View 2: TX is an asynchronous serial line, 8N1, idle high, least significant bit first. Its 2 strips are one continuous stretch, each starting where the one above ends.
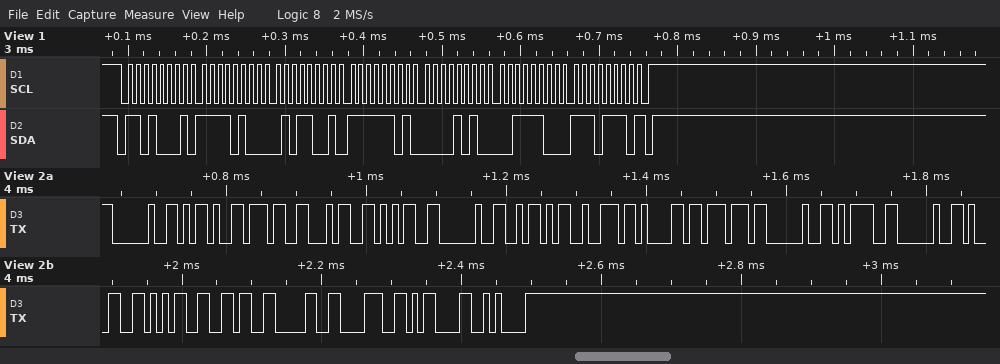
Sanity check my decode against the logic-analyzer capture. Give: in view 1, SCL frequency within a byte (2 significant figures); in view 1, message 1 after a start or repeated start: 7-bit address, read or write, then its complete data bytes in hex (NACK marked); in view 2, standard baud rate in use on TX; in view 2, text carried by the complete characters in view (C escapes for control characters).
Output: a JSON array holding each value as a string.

["100 kHz", "0x68 read: F4 59 FD 0A 3C EE NACK", "115200 baud", "\" -745 Zraw = 15608\\r\\n\""]
